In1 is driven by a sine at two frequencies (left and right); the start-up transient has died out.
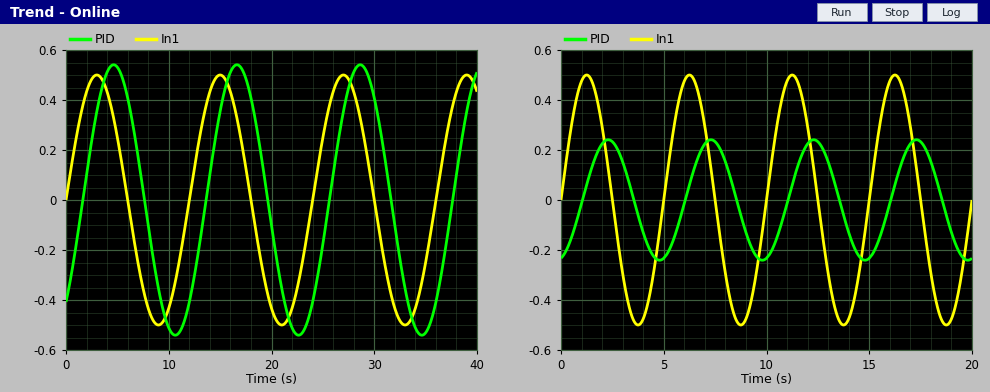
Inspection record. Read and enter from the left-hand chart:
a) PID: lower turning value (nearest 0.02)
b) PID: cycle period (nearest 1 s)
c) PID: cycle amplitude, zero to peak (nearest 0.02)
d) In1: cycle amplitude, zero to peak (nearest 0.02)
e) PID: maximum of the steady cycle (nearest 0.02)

-0.54
12 s
0.54
0.50
0.54
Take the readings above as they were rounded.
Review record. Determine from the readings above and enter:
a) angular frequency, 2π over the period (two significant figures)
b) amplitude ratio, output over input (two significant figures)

0.52 rad/s
1.1
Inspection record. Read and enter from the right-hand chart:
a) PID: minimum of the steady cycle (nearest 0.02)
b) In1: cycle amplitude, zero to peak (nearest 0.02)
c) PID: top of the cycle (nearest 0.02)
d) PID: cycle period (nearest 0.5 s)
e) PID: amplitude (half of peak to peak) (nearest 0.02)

-0.24
0.50
0.24
5.0 s
0.24
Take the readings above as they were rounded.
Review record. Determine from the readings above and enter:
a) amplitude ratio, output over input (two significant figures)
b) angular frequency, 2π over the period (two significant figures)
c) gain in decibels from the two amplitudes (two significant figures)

0.48
1.3 rad/s
-6.4 dB
